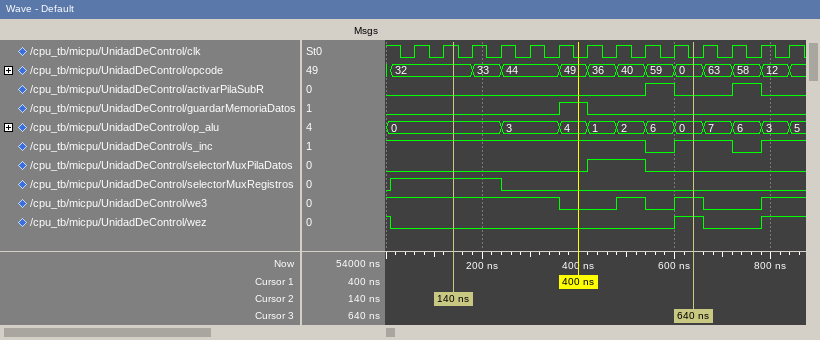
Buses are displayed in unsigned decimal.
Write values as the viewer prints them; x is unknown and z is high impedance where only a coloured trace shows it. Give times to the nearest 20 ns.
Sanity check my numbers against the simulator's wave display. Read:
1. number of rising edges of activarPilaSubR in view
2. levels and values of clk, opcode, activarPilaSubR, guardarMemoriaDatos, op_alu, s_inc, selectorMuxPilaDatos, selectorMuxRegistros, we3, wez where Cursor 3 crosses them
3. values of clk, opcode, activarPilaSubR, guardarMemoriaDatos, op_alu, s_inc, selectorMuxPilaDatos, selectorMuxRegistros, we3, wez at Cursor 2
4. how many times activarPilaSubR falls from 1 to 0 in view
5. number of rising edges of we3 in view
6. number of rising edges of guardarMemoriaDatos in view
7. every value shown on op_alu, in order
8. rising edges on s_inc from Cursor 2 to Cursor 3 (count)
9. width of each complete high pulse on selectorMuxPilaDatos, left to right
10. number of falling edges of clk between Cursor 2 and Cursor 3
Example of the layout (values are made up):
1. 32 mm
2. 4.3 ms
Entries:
1. 2
2. clk=0, opcode=0, activarPilaSubR=0, guardarMemoriaDatos=0, op_alu=0, s_inc=1, selectorMuxPilaDatos=0, selectorMuxRegistros=0, we3=1, wez=1
3. clk=1, opcode=32, activarPilaSubR=0, guardarMemoriaDatos=0, op_alu=0, s_inc=1, selectorMuxPilaDatos=0, selectorMuxRegistros=1, we3=1, wez=0
4. 2
5. 3
6. 1
7. 0, 3, 4, 1, 2, 6, 0, 7, 6, 3, 5
8. 1
9. 120 ns
10. 9
